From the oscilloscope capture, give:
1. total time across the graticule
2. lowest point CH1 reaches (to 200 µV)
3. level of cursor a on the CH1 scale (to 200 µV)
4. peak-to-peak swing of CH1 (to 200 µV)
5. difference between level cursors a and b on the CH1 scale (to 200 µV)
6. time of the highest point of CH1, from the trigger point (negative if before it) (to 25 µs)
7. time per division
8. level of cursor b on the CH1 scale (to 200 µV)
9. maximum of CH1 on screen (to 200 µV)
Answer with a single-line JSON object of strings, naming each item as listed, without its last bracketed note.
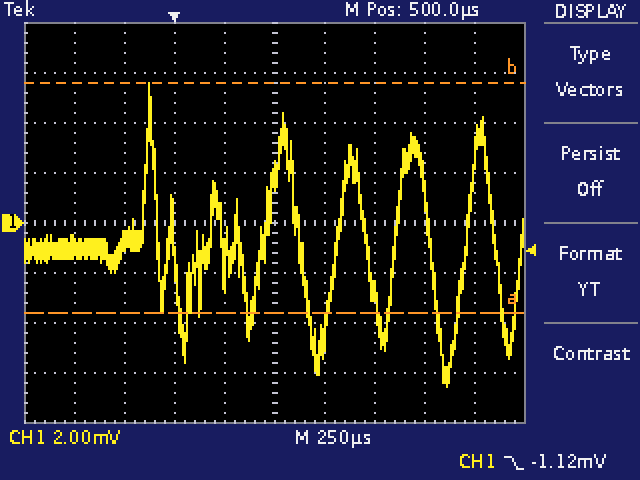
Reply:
{"total time across the graticule": "2.5 ms", "lowest point CH1 reaches": "-6.6 mV", "level of cursor a on the CH1 scale": "-3.6 mV", "peak-to-peak swing of CH1": "12.2 mV", "difference between level cursors a and b on the CH1 scale": "9.2 mV", "time of the highest point of CH1, from the trigger point (negative if before it)": "-125 µs", "time per division": "250 µs", "level of cursor b on the CH1 scale": "5.6 mV", "maximum of CH1 on screen": "5.6 mV"}
